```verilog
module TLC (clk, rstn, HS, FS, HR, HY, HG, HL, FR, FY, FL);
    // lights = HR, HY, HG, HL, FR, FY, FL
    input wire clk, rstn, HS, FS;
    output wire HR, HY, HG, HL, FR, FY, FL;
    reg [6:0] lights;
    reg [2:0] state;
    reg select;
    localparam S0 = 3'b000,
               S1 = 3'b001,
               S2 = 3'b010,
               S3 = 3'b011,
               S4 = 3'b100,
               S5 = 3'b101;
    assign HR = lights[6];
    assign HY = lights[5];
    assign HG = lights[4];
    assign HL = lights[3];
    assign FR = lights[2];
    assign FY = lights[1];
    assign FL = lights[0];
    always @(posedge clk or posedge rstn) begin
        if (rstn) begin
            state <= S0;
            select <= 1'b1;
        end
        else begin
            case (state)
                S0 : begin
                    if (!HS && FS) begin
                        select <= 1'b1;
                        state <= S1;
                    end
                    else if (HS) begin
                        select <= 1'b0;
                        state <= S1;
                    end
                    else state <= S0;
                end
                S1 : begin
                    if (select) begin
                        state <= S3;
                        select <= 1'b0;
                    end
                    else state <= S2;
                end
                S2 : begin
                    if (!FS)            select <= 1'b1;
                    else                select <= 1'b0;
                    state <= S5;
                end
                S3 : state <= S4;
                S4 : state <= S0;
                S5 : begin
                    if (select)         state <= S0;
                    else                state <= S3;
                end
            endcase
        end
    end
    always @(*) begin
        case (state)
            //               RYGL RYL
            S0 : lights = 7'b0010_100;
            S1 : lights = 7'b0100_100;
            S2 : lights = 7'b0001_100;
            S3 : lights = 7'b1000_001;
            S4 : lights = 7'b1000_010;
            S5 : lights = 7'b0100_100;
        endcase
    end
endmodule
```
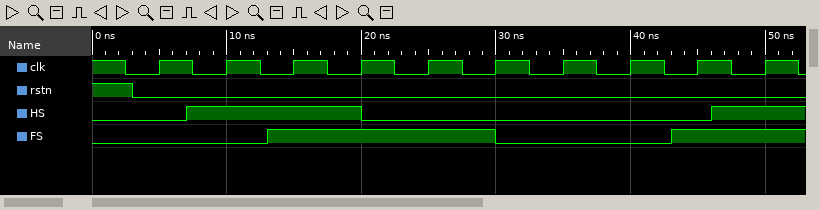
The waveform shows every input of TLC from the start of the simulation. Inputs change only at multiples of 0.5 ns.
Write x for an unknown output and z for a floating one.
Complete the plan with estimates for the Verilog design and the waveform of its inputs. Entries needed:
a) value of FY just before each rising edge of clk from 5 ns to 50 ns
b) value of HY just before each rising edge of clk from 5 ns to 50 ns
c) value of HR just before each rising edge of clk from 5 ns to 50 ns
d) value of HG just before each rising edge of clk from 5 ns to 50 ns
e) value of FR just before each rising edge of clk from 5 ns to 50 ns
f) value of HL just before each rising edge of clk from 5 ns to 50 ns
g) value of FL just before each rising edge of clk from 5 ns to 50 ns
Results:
0 0 0 0 0 0 1 0 0 0
0 0 1 0 1 0 0 0 0 1
0 0 0 0 0 1 1 0 0 0
1 1 0 0 0 0 0 1 1 0
1 1 1 1 1 0 0 1 1 1
0 0 0 1 0 0 0 0 0 0
0 0 0 0 0 1 0 0 0 0
